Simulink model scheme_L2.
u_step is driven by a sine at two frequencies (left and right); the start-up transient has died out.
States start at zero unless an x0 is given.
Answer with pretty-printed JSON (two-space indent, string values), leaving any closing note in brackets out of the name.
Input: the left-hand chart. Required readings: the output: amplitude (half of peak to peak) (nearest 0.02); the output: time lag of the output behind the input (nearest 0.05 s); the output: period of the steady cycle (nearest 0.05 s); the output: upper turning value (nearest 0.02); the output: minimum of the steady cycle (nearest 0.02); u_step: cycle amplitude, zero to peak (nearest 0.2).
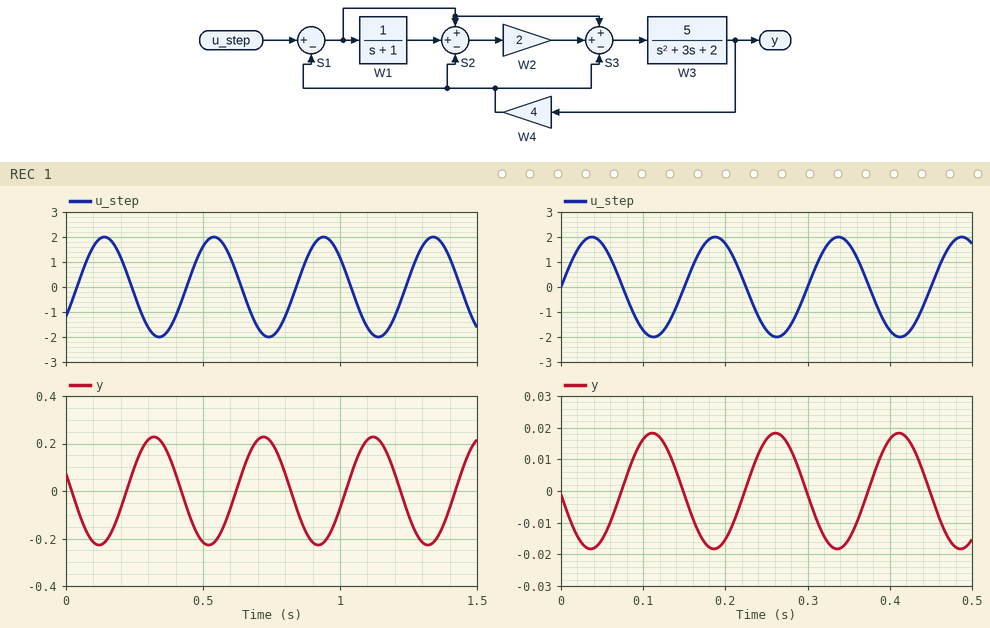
{
  "the output: amplitude (half of peak to peak)": "0.22",
  "the output: time lag of the output behind the input": "0.20 s",
  "the output: period of the steady cycle": "0.40 s",
  "the output: upper turning value": "0.22",
  "the output: minimum of the steady cycle": "-0.22",
  "u_step: cycle amplitude, zero to peak": "2.0"
}
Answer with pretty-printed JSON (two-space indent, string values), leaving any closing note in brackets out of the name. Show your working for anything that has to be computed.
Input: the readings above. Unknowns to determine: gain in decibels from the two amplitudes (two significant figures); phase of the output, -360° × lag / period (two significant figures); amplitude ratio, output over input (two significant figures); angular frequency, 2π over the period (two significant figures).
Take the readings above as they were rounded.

{
  "gain in decibels from the two amplitudes": "20 log10(0.22 / 2) = -19 dB",
  "phase of the output, -360° × lag / period": "-360 × 0.2 / 0.4 = -180°",
  "amplitude ratio, output over input": "0.22 / 2 = 0.11",
  "angular frequency, 2π over the period": "2π / 0.4 = 16 rad/s"
}
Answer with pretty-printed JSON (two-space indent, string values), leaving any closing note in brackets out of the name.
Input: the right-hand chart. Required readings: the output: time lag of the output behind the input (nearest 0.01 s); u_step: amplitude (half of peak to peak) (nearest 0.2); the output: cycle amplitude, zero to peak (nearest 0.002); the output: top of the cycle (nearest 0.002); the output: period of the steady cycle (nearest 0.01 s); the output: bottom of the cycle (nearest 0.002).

{
  "the output: time lag of the output behind the input": "0.07 s",
  "u_step: amplitude (half of peak to peak)": "2.0",
  "the output: cycle amplitude, zero to peak": "0.018",
  "the output: top of the cycle": "0.018",
  "the output: period of the steady cycle": "0.15 s",
  "the output: bottom of the cycle": "-0.018"
}
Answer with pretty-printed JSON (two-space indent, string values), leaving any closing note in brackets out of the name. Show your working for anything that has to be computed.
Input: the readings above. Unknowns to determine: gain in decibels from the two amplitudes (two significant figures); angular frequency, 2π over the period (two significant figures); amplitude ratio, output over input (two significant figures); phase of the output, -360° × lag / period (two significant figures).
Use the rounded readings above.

{
  "gain in decibels from the two amplitudes": "20 log10(0.018 / 2) = -41 dB",
  "angular frequency, 2π over the period": "2π / 0.15 = 42 rad/s",
  "amplitude ratio, output over input": "0.018 / 2 = 0.0090",
  "phase of the output, -360° × lag / period": "-360 × 0.07 / 0.15 = -170°"
}
